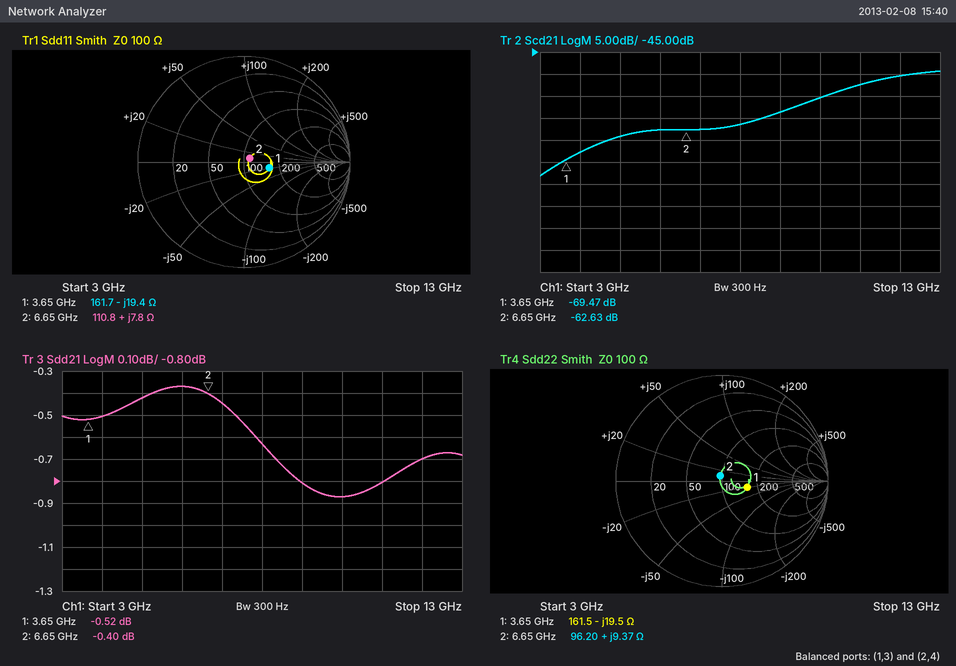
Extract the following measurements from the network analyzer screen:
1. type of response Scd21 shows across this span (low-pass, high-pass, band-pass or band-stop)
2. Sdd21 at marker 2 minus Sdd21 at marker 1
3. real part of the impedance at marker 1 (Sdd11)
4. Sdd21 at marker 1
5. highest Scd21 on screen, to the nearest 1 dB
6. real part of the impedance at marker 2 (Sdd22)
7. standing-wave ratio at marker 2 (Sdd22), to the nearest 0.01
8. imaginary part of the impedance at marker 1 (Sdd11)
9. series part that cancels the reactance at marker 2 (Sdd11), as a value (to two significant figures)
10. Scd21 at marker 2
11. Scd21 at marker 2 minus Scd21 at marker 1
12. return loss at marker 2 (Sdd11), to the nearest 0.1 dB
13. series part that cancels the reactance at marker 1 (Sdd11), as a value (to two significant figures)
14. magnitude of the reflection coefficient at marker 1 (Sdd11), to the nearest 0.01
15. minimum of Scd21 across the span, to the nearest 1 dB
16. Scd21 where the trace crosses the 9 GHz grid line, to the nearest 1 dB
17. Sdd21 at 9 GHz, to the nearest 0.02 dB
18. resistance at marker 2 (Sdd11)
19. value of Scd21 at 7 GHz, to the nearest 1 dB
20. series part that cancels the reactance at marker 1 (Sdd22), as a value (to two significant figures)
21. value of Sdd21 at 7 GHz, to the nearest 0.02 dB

high-pass
0.12 dB
161.7 Ω
-0.52 dB
-49 dB
96.20 Ω
1.11
-19.4 Ω
3.1 pF
-62.63 dB
6.84 dB
24.0 dB
850 pH
0.25
-73 dB
-59 dB
-0.80 dB
110.8 Ω
-63 dB
850 pH
-0.44 dB
